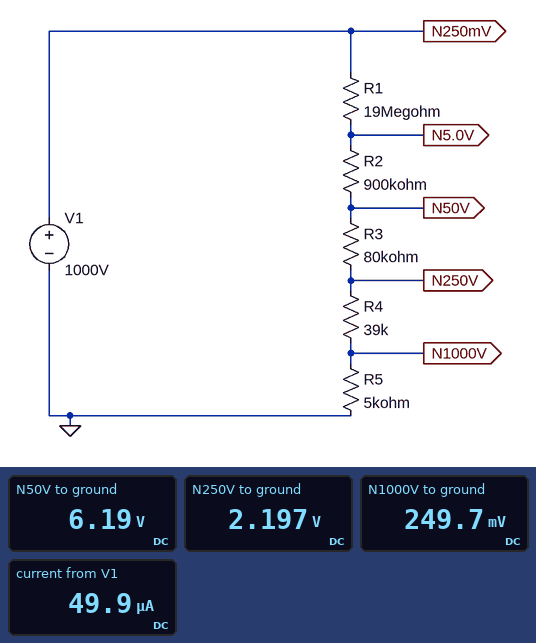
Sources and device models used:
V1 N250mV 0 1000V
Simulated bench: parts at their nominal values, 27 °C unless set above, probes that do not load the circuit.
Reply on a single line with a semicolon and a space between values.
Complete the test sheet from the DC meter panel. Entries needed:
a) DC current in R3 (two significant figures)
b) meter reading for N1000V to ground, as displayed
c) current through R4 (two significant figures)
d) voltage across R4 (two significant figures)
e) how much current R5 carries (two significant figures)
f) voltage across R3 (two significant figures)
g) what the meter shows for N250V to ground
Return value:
50 µA; 249.7 mV; 50 µA; 1.9 V; 50 µA; 4.0 V; 2.197 V
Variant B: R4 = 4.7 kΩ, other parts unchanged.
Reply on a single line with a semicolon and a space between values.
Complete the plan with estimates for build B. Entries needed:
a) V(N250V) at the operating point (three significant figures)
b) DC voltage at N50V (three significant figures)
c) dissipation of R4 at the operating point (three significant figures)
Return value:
485 mV; 4.49 V; 11.8 µW
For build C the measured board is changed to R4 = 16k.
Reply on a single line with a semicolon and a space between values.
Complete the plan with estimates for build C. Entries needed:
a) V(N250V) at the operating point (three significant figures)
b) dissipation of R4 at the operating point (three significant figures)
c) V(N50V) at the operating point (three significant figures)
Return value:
1.05 V; 40.0 µW; 5.05 V
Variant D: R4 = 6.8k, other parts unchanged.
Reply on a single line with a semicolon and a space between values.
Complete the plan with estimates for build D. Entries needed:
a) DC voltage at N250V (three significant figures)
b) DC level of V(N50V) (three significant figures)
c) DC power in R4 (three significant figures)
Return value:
590 mV; 4.59 V; 17.0 µW
